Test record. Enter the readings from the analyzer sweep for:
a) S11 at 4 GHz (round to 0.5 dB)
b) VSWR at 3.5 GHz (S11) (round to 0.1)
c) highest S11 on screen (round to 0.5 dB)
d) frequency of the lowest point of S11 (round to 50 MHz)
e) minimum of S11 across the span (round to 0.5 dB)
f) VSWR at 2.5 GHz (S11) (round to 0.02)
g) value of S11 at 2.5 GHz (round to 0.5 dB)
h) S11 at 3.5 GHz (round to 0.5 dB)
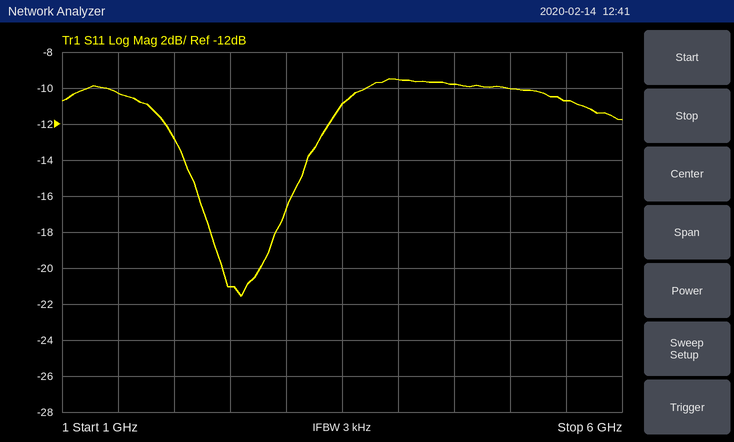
-9.5 dB
1.8
-9.5 dB
2.60 GHz
-21.5 dB
1.20
-21.0 dB
-11.0 dB
